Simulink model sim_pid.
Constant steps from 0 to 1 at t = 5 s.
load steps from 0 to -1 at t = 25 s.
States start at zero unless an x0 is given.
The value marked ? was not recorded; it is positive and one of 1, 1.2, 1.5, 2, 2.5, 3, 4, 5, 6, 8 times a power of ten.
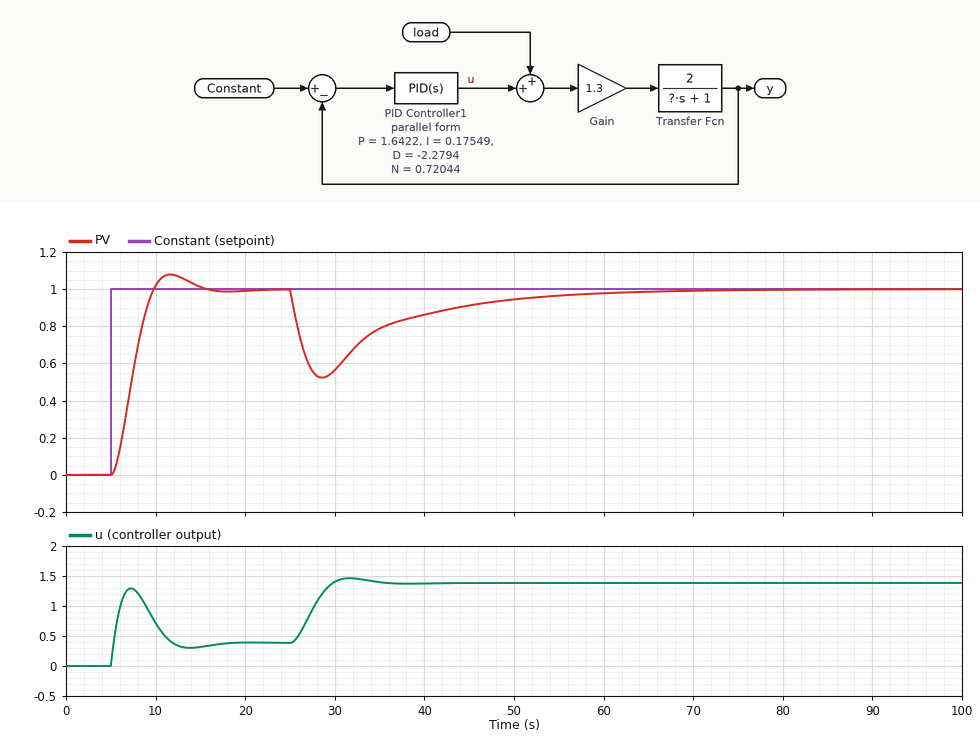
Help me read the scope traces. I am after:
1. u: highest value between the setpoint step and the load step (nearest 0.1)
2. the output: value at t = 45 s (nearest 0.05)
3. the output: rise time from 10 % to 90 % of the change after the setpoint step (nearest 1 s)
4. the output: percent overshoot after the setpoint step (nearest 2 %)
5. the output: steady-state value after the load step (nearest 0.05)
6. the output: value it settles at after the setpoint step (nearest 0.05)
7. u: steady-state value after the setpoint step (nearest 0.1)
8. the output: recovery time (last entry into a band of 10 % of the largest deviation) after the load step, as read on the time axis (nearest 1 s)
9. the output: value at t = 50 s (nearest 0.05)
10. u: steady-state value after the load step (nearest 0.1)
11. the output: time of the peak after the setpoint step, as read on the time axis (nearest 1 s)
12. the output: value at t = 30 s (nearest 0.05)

1.3
0.90
3 s
8 %
1.00
1.00
0.4
52 s
0.95
1.4
12 s
0.55
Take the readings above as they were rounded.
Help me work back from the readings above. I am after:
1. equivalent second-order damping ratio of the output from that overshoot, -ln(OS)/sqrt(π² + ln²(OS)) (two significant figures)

0.63
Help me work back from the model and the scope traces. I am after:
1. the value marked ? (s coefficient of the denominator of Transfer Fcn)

10
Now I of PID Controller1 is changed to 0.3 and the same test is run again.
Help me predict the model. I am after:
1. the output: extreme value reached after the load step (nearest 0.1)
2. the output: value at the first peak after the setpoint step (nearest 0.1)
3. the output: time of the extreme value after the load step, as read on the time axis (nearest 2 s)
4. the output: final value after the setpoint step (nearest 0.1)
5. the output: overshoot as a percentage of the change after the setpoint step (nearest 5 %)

0.6
1.2
28 s
1.0
20 %
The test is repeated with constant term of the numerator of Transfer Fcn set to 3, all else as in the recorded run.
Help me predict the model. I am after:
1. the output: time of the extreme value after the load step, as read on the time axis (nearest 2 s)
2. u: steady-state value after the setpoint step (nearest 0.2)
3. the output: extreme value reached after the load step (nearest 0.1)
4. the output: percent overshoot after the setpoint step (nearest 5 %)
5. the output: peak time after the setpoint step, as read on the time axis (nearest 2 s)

28 s
0.2
0.4
15 %
10 s
